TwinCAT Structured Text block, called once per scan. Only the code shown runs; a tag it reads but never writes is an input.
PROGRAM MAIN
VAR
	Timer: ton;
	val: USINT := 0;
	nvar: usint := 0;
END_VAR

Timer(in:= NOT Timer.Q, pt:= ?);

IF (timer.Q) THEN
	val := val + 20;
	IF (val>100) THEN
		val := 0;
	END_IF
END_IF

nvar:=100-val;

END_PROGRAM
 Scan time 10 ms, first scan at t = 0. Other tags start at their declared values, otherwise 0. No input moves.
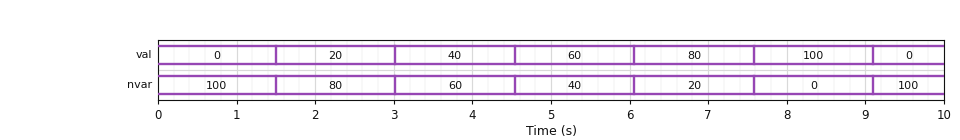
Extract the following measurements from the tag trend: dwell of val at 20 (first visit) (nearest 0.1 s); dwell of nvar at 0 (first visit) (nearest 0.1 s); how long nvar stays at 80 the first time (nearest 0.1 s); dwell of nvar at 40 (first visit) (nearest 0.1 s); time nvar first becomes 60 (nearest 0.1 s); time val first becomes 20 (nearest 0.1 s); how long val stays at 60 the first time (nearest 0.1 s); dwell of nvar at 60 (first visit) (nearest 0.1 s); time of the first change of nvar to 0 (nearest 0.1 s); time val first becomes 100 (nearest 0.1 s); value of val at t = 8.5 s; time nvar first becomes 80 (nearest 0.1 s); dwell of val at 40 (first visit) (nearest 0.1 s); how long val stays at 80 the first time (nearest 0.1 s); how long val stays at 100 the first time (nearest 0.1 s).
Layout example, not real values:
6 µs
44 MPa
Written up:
1.5 s
1.5 s
1.5 s
1.5 s
3.0 s
1.5 s
1.5 s
1.5 s
7.6 s
7.6 s
100
1.5 s
1.5 s
1.5 s
1.5 s
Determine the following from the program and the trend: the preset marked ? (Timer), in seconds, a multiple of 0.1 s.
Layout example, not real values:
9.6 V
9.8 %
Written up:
1.5 s
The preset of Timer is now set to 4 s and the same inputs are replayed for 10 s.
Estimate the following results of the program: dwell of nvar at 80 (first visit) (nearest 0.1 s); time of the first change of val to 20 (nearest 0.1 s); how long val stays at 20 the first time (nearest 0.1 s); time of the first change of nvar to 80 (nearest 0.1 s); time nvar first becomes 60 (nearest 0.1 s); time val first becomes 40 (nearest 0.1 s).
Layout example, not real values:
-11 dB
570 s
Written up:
4.0 s
4.0 s
4.0 s
4.0 s
8.0 s
8.0 s
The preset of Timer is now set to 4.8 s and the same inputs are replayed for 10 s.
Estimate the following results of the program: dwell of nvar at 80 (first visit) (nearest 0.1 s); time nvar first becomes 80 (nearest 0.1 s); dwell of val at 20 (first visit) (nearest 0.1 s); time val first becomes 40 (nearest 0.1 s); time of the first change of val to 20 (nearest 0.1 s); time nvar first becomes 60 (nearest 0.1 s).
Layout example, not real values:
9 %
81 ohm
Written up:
4.8 s
4.8 s
4.8 s
9.6 s
4.8 s
9.6 s
